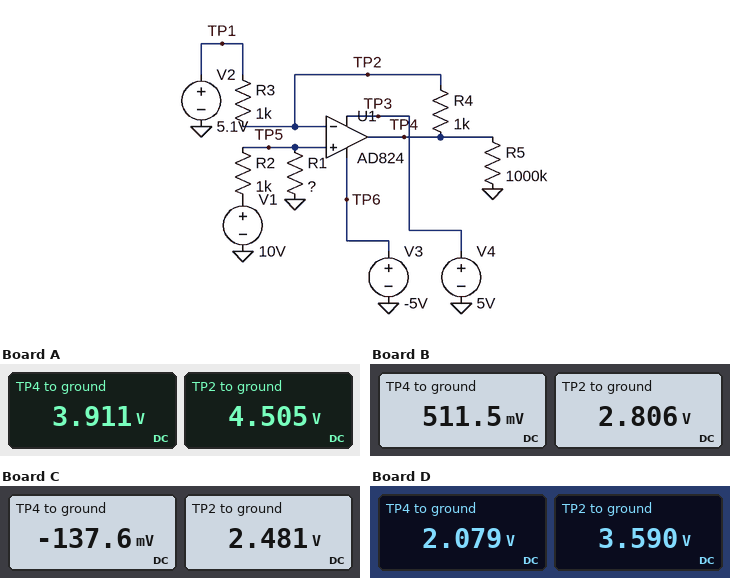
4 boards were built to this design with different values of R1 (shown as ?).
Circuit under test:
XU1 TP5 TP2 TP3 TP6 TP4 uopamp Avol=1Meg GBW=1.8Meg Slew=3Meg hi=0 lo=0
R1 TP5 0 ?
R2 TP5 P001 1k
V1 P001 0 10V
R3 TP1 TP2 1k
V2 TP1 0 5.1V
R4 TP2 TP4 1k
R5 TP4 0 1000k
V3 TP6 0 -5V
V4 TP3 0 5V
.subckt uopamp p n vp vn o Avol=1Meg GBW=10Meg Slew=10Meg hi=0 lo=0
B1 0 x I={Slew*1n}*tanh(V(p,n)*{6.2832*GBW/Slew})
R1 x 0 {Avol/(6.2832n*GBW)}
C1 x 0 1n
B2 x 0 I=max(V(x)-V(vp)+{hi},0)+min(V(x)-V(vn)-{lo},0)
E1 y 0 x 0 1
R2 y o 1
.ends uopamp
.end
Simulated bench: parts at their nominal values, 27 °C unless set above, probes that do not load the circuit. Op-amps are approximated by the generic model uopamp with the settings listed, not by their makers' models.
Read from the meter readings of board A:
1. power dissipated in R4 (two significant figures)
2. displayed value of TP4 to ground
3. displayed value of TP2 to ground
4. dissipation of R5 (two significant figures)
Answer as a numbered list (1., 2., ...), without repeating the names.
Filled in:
1. 350 µW
2. 3.911 V
3. 4.505 V
4. 15 µW
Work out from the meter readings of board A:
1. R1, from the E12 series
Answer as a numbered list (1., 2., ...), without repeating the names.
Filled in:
1. 820 Ω
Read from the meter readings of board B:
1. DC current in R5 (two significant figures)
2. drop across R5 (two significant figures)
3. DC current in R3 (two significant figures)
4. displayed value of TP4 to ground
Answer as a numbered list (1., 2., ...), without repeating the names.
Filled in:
1. 510 nA
2. 510 mV
3. 2.3 mA
4. 511.5 mV
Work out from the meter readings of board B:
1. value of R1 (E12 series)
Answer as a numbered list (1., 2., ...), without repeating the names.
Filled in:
1. 390 Ω
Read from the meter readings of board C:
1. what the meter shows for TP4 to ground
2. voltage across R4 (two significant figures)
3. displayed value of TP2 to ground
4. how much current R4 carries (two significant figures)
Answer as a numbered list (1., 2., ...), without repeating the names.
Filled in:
1. -137.6 mV
2. 2.6 V
3. 2.481 V
4. 2.6 mA
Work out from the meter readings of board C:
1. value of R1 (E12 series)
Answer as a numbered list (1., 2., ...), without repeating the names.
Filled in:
1. 330 Ω
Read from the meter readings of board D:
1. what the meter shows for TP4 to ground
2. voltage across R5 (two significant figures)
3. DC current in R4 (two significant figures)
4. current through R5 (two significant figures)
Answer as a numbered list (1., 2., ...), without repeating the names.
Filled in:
1. 2.079 V
2. 2.1 V
3. 1.5 mA
4. 2.1 µA
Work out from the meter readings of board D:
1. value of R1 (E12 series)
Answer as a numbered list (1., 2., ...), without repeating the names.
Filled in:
1. 560 Ω
